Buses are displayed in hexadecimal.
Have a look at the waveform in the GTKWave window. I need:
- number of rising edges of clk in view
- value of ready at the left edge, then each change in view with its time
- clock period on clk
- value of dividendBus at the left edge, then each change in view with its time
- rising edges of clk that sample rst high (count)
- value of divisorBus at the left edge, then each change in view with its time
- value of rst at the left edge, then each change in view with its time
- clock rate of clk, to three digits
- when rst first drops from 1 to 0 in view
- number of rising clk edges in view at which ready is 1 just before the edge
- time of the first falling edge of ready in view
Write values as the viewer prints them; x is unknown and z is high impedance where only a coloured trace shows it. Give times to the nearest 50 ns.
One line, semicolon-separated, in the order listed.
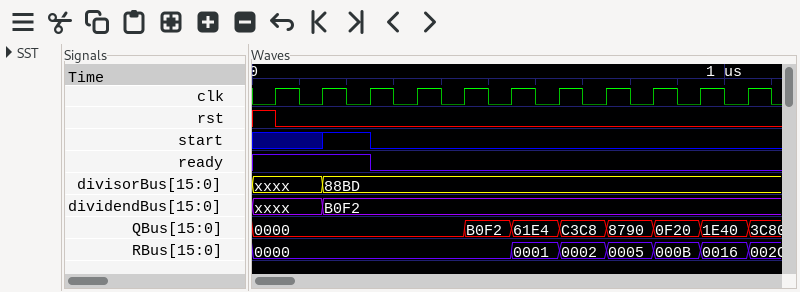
11; 1, 0 at 250 ns; 100 ns; xxxx, B0F2 at 150 ns; 1; xxxx, 88BD at 150 ns; 1, 0 at 50 ns; 10.0 MHz; 50 ns; 3; 250 ns
